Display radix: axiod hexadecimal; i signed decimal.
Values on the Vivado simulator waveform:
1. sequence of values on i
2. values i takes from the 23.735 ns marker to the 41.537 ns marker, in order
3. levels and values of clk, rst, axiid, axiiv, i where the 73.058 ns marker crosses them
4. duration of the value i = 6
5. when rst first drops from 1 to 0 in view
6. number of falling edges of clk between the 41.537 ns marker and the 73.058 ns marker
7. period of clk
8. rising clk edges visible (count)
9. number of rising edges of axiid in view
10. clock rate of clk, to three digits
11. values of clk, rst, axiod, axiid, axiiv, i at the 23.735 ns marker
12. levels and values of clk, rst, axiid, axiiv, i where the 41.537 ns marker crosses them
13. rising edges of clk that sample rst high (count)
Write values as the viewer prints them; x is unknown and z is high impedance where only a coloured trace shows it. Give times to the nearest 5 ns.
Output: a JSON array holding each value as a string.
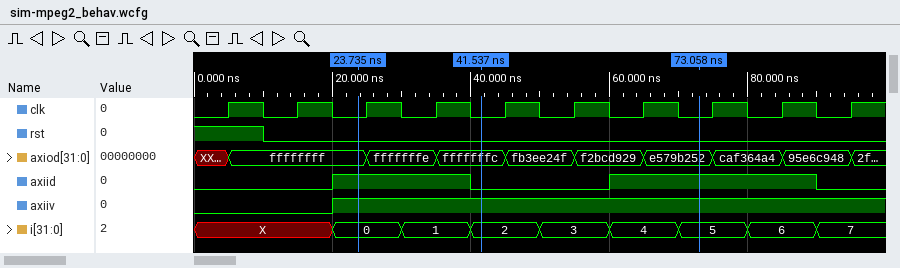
["X, 0, 1, 2, 3, 4, 5, 6, 7", "0, 1, 2", "clk=0, rst=0, axiid=1, axiiv=1, i=5", "10 ns", "10 ns", "3", "10 ns", "10", "2", "100 MHz", "clk=0, rst=0, axiod=ffffffff, axiid=1, axiiv=1, i=0", "clk=0, rst=0, axiid=0, axiiv=1, i=2", "1"]
